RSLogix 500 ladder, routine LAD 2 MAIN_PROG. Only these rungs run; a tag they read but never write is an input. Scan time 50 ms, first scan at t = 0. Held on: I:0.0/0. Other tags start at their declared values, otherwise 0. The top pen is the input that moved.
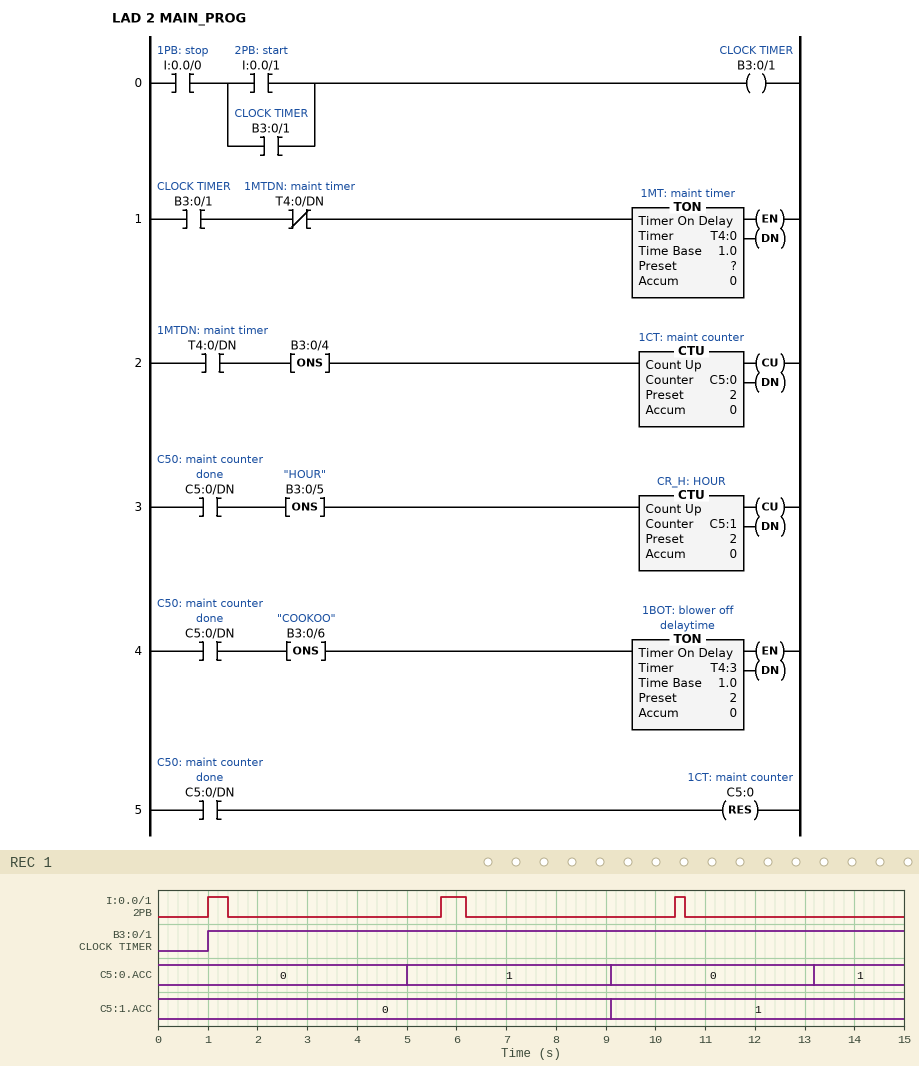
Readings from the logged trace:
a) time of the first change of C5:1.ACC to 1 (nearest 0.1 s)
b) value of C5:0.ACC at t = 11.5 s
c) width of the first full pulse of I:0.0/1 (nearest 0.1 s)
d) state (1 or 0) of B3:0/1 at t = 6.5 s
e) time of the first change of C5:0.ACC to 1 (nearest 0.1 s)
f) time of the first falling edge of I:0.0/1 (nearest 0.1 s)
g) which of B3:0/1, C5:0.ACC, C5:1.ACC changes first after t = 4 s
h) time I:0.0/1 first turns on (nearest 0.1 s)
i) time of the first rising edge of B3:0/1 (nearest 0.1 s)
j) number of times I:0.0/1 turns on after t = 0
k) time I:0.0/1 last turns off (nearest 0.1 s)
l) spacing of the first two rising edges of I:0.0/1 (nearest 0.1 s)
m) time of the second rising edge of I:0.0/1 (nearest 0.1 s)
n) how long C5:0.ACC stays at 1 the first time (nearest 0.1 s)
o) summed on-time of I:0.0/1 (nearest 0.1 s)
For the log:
9.1 s
0
0.4 s
1
5.0 s
1.4 s
C5:0.ACC
1.0 s
1.0 s
3
10.6 s
4.7 s
5.7 s
4.1 s
1.1 s
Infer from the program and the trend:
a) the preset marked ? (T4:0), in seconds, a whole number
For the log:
4 s
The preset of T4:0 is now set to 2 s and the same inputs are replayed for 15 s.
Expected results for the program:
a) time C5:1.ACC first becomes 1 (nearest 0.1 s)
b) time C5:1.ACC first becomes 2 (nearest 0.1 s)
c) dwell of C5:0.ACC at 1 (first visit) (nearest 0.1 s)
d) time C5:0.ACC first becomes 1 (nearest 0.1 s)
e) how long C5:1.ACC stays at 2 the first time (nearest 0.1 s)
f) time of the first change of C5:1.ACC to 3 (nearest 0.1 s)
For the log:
5.1 s
9.3 s
2.1 s
3.0 s
4.2 s
13.5 s
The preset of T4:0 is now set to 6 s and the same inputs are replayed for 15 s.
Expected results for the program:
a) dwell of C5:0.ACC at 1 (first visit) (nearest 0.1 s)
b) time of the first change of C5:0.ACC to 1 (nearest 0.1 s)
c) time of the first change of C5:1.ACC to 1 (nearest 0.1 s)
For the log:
6.1 s
7.0 s
13.1 s
